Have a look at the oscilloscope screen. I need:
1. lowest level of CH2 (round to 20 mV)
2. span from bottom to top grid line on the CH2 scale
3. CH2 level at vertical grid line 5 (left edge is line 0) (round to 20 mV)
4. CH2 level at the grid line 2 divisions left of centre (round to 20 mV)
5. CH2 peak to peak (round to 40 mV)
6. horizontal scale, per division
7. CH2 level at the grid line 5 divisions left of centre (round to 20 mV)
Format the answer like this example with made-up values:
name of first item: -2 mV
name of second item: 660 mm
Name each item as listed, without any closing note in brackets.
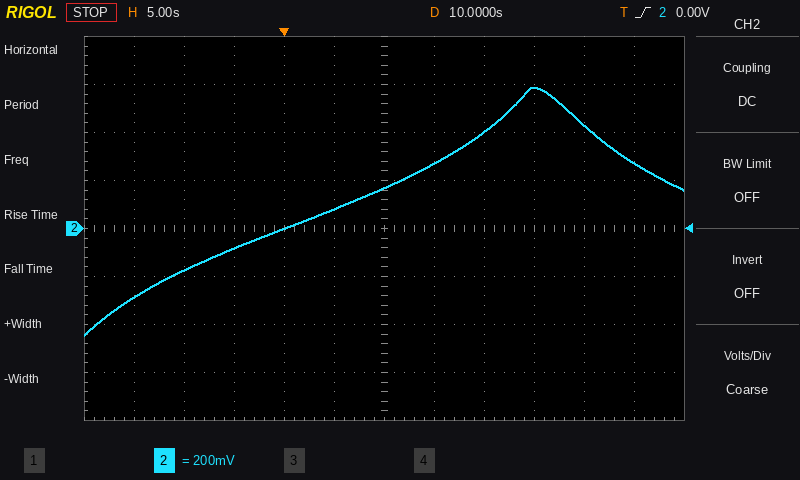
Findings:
lowest level of CH2: -440 mV
span from bottom to top grid line on the CH2 scale: 1.6 V
CH2 level at vertical grid line 5 (left edge is line 0): 80 mV
CH2 level at the grid line 2 divisions left of centre: 0 mV
CH2 peak to peak: 1.04 V
horizontal scale, per division: 5 s
CH2 level at the grid line 5 divisions left of centre: -280 mV
